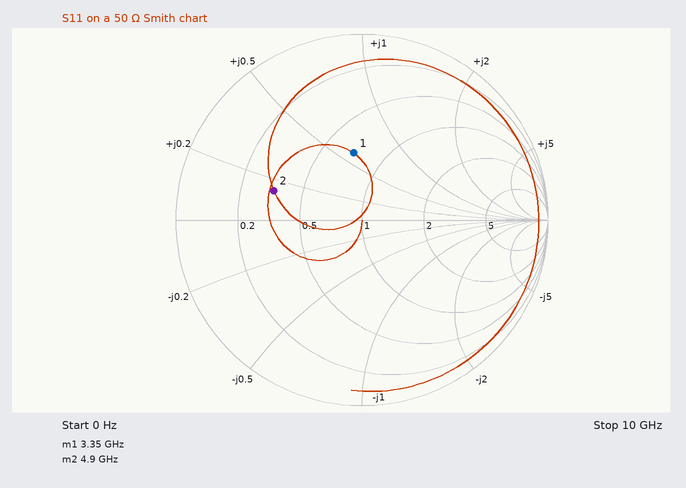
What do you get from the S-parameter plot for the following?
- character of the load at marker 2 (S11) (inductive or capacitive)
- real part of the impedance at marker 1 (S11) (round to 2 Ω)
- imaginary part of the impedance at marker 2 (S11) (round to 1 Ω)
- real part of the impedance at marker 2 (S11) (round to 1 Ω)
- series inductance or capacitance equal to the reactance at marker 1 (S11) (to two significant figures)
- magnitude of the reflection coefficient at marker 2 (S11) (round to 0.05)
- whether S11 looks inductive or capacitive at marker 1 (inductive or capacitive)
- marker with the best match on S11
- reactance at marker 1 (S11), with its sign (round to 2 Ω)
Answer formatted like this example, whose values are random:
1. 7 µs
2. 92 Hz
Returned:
1. inductive
2. 36 Ω
3. +7 Ω
4. 17 Ω
5. 1.4 nH
6. 0.50
7. inductive
8. marker 1
9. +30 Ω
